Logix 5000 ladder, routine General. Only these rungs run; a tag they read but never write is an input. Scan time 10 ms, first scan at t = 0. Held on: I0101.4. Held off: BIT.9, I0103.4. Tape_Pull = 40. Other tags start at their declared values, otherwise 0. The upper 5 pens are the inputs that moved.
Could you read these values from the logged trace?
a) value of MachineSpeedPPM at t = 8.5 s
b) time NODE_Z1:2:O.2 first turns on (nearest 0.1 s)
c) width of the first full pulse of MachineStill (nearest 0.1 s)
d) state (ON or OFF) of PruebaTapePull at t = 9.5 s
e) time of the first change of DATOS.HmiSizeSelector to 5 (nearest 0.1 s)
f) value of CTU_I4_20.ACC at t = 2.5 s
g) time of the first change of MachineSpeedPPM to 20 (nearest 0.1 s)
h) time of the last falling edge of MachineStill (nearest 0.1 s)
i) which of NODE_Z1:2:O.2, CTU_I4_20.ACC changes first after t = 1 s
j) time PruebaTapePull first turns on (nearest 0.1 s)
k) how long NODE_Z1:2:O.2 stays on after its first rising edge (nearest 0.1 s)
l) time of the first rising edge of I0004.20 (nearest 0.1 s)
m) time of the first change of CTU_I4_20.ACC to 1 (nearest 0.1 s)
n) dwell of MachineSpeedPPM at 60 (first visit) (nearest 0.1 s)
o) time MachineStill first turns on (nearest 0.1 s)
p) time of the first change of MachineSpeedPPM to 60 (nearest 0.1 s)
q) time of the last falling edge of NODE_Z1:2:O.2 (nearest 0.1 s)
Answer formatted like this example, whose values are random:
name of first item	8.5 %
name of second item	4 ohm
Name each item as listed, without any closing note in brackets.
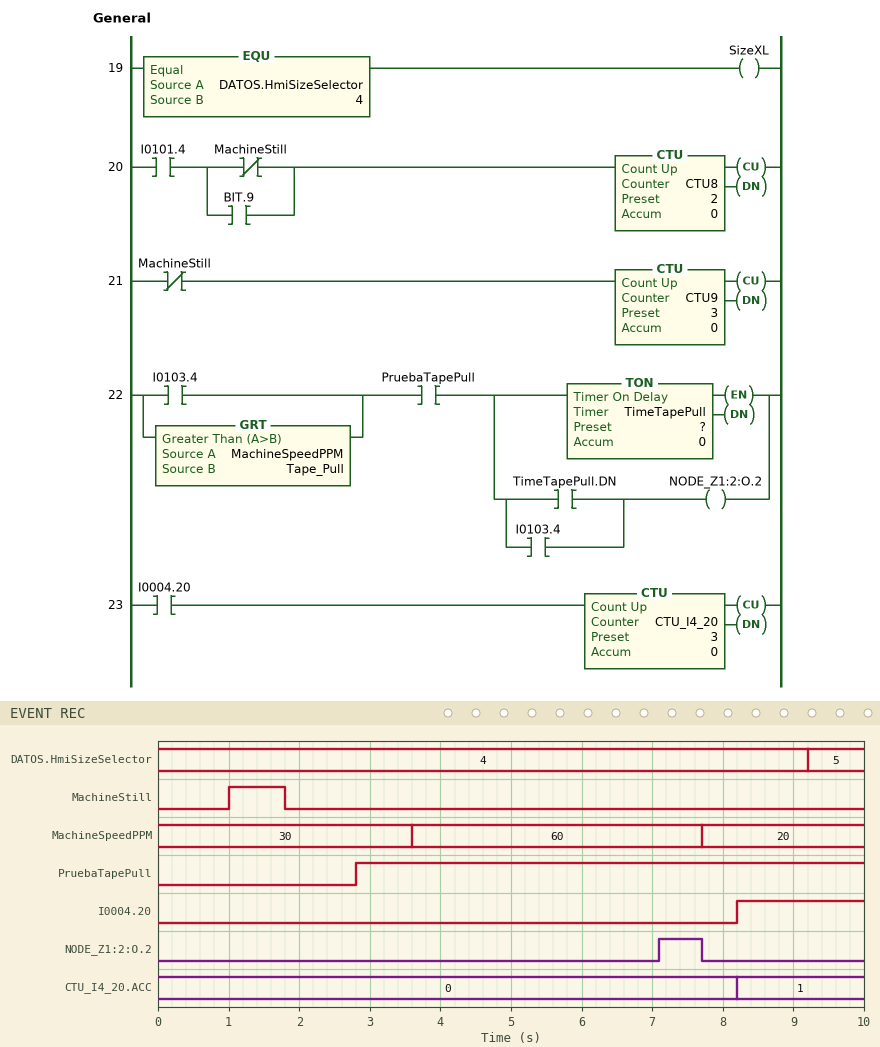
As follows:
value of MachineSpeedPPM at t = 8.5 s	20
time NODE_Z1:2:O.2 first turns on	7.1 s
width of the first full pulse of MachineStill	0.8 s
state (ON or OFF) of PruebaTapePull at t = 9.5 s	ON
time of the first change of DATOS.HmiSizeSelector to 5	9.2 s
value of CTU_I4_20.ACC at t = 2.5 s	0
time of the first change of MachineSpeedPPM to 20	7.7 s
time of the last falling edge of MachineStill	1.8 s
which of NODE_Z1:2:O.2, CTU_I4_20.ACC changes first after t = 1 s	NODE_Z1:2:O.2
time PruebaTapePull first turns on	2.8 s
how long NODE_Z1:2:O.2 stays on after its first rising edge	0.6 s
time of the first rising edge of I0004.20	8.2 s
time of the first change of CTU_I4_20.ACC to 1	8.2 s
dwell of MachineSpeedPPM at 60 (first visit)	4.1 s
time MachineStill first turns on	1.0 s
time of the first change of MachineSpeedPPM to 60	3.6 s
time of the last falling edge of NODE_Z1:2:O.2	7.7 s
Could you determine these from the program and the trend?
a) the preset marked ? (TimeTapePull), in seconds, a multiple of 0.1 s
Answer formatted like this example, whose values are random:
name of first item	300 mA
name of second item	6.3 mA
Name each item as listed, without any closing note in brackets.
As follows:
the preset marked ? (TimeTapePull), in seconds, a multiple of 0.1 s	3.5 s
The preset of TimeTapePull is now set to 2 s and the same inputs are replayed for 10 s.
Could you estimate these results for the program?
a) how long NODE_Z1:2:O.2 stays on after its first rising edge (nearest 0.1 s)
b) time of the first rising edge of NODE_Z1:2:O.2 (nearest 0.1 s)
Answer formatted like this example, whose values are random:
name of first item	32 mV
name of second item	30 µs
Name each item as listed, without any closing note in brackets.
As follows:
how long NODE_Z1:2:O.2 stays on after its first rising edge	2.1 s
time of the first rising edge of NODE_Z1:2:O.2	5.6 s
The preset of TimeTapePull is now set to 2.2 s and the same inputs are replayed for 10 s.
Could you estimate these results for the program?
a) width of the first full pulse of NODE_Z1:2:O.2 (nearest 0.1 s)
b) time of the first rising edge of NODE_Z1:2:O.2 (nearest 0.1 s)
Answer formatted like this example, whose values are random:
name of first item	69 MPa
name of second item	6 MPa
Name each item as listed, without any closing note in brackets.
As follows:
width of the first full pulse of NODE_Z1:2:O.2	1.9 s
time of the first rising edge of NODE_Z1:2:O.2	5.8 s
